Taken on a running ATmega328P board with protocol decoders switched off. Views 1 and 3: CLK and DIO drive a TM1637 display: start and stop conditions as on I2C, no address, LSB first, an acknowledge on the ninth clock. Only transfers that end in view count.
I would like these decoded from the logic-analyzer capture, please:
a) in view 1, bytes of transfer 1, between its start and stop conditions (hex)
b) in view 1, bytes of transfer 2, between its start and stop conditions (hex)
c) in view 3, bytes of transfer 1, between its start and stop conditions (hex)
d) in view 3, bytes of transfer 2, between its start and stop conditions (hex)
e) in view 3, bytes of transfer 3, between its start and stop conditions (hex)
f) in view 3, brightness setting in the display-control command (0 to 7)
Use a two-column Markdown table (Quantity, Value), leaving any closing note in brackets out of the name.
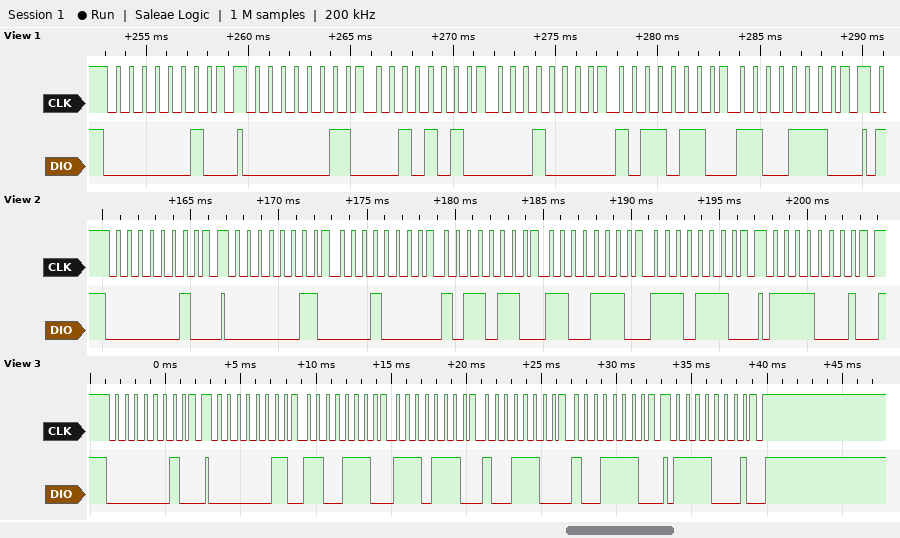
| Quantity | Value |
|---|---|
| in view 1, bytes of transfer 1, between its start and stop conditions | 40 |
| in view 1, bytes of transfer 2, between its start and stop conditions | C0 54 08 6D 73 |
| in view 3, bytes of transfer 1, between its start and stop conditions | 40 |
| in view 3, bytes of transfer 2, between its start and stop conditions | C0 73 77 39 79 |
| in view 3, bytes of transfer 3, between its start and stop conditions | 8F |
| in view 3, brightness setting in the display-control command | 7 |
